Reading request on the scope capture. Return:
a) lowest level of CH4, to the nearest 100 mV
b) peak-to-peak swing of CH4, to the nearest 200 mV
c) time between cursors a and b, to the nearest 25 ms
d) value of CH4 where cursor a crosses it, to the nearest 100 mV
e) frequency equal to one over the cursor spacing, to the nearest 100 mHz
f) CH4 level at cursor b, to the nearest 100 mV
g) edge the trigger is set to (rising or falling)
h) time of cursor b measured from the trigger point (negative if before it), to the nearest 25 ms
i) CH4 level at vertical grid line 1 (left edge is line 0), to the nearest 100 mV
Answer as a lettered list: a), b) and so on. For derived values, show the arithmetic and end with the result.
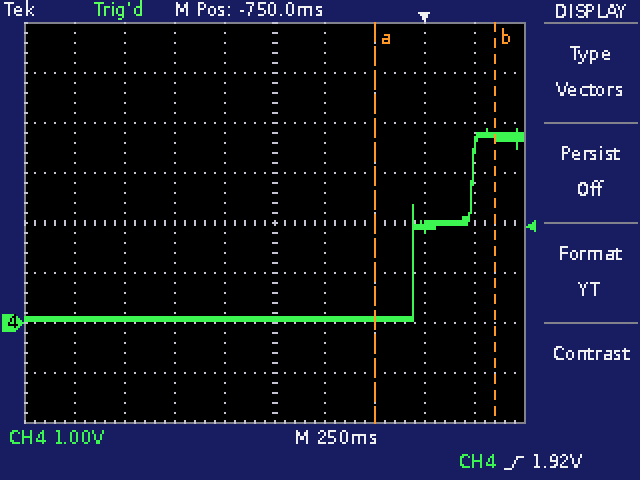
a) 0.0 V
b) 3.8 V
c) 600 ms
d) 100 mV
e) 1 / 600 ms ≈ 1.7 Hz
f) 3.7 V
g) rising
h) +350 ms
i) 100 mV
